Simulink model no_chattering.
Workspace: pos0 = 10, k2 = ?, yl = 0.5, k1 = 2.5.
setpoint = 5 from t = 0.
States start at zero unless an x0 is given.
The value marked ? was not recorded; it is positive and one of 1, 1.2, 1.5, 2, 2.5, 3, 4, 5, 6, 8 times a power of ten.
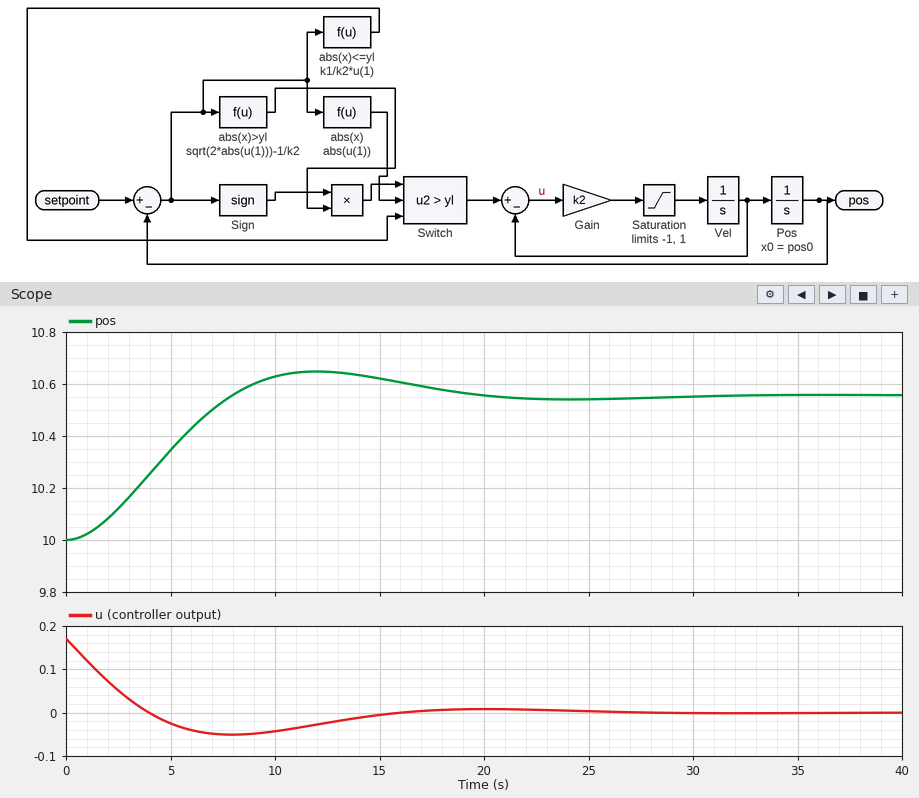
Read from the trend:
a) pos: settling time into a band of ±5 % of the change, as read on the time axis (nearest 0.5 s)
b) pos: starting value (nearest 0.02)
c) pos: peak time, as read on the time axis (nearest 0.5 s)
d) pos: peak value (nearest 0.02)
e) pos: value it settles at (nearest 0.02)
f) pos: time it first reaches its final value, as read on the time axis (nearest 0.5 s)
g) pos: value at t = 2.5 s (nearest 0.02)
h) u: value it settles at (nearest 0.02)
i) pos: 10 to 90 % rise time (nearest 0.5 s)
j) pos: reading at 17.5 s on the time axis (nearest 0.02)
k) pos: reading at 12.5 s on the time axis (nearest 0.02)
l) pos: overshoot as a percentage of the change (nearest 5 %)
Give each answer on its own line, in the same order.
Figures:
17.5 s
10.00
12.0 s
10.64
10.56
8.0 s
10.12
0.00
5.5 s
10.58
10.64
15 %
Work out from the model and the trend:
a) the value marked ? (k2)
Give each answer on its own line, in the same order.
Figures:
0.3
